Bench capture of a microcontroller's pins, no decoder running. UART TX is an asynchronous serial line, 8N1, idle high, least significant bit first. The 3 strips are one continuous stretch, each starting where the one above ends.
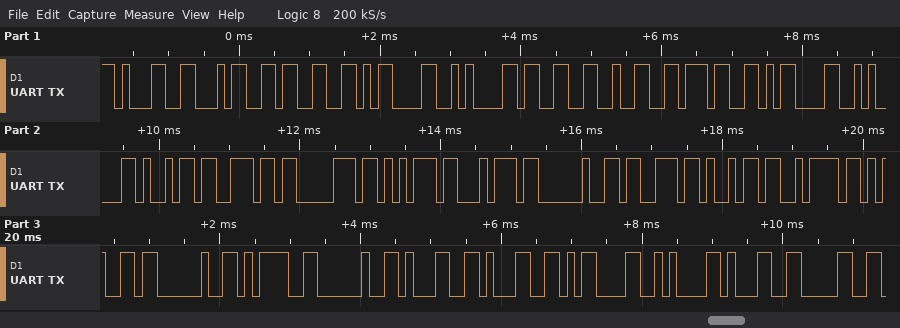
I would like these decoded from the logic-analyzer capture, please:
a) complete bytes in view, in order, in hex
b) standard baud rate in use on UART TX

31 34 33 0D 0A 33 32 37 0D 0A 69 6E 70 75 74 20 73 69 7A 65 20 3D 20 31 31 0D 0A 31 30
9600 baud
